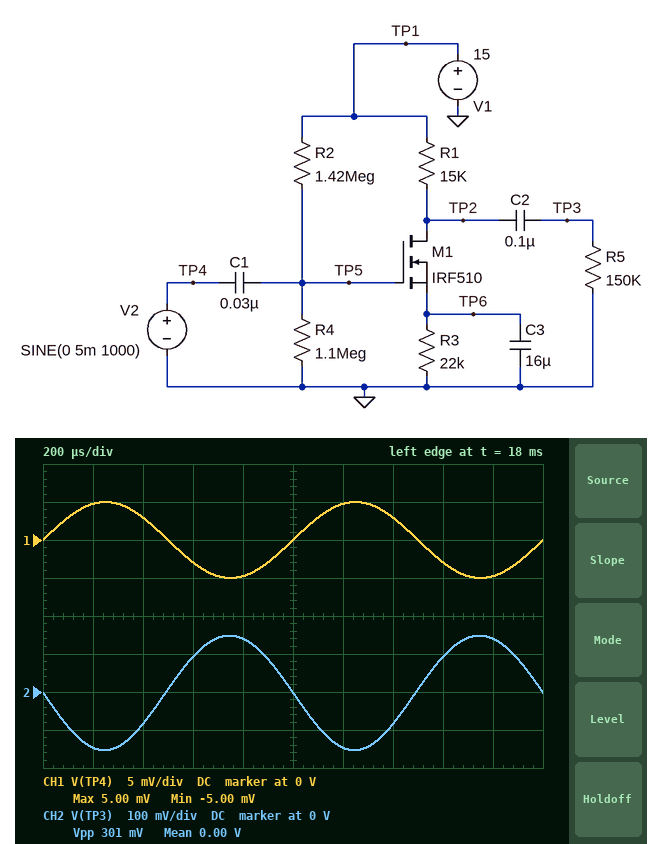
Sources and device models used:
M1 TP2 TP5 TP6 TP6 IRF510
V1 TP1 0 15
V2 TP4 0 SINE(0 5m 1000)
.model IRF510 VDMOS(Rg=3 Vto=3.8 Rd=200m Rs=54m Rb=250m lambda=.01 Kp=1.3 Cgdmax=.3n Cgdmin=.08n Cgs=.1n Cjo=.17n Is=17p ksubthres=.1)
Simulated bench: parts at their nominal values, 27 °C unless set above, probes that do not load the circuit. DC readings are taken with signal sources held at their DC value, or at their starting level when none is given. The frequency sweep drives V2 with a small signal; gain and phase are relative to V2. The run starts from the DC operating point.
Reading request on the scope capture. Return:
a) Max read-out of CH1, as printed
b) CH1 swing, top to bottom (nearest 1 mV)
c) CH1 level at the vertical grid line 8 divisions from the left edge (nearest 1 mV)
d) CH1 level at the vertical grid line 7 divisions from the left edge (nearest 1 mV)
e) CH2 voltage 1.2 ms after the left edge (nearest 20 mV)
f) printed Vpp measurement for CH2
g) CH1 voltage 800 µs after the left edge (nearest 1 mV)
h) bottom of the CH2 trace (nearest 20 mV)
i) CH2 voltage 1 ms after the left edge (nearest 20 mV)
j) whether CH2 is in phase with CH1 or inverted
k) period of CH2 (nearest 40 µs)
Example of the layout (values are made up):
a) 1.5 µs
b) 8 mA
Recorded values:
a) 5.00 mV
b) 10 mV
c) -3 mV
d) 3 mV
e) -140 mV
f) 301 mV
g) -5 mV
h) -160 mV
i) 0 V
j) inverted
k) 1.00 ms
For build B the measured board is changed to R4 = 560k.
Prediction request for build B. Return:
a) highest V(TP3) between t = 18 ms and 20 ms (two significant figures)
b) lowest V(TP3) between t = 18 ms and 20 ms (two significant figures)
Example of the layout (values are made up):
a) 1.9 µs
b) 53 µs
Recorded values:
a) 40 mV
b) -42 mV
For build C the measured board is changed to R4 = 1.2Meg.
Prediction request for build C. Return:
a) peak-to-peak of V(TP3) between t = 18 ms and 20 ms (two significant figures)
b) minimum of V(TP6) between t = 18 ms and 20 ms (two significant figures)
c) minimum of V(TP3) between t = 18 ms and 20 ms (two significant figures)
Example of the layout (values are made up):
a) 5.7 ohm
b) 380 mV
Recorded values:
a) 330 mV
b) 3.3 V
c) -170 mV
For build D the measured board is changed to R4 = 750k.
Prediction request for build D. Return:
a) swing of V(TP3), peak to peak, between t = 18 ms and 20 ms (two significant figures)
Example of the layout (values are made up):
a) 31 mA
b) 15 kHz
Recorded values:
a) 180 mV
